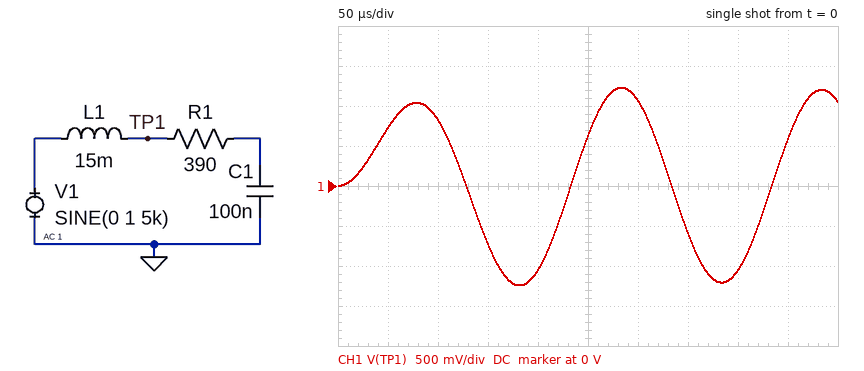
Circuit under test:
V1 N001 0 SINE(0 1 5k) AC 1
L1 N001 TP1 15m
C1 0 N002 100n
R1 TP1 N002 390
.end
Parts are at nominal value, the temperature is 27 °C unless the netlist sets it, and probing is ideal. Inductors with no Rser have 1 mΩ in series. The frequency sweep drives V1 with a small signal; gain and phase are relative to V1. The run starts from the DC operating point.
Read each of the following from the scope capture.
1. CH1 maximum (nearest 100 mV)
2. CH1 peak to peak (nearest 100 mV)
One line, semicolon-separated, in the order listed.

1.2 V; 2.5 V
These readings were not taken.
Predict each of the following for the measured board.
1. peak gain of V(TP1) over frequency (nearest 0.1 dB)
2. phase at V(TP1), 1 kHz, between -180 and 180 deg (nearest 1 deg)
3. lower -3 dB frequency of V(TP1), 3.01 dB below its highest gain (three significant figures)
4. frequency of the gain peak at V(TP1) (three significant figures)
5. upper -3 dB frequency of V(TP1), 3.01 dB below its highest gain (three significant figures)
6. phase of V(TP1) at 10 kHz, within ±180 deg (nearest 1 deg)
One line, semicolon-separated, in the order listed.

3.3 dB; -1 deg; 763 Hz; 3.51 kHz; 5.66 kHz; -86 deg
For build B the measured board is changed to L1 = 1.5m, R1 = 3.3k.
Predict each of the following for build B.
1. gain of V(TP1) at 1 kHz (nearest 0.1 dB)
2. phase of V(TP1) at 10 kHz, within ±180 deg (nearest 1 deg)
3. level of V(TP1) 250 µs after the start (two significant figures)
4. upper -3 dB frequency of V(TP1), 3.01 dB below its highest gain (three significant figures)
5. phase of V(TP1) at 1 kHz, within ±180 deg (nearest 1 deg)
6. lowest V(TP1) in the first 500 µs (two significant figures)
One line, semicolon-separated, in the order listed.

0 dB; -2 deg; 1.0 V; 350 kHz; 0 deg; -1.0 V
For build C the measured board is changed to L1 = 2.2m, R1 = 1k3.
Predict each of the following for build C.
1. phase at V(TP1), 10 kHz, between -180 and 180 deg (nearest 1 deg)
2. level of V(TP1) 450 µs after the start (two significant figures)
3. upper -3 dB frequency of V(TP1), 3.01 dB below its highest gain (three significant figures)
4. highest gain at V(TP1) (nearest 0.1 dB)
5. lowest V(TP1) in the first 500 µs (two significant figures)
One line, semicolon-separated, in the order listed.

-6 deg; 1.0 V; 93.2 kHz; 0.1 dB; -1.0 V
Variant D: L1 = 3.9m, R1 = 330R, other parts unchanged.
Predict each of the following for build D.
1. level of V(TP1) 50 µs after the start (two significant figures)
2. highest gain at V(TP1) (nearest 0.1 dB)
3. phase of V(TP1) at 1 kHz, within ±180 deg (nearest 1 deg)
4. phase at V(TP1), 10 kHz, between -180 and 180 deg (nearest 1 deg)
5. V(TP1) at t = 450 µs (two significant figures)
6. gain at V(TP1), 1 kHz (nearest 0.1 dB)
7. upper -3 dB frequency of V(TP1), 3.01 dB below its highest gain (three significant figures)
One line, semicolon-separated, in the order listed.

1.1 V; 1.6 dB; 0 deg; -40 deg; 1.2 V; 0.1 dB; 14.3 kHz
